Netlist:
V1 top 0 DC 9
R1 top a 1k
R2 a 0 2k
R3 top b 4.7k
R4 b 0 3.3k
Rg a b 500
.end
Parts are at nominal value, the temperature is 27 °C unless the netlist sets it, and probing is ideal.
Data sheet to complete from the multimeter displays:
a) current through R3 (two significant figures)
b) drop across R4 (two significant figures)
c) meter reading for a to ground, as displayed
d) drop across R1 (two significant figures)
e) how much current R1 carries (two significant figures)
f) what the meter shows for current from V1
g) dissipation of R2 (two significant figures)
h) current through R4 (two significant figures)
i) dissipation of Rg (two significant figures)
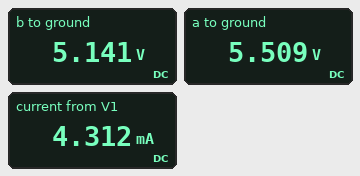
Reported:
820 µA
5.1 V
5.509 V
3.5 V
3.5 mA
4.312 mA
15 mW
1.6 mA
270 µW
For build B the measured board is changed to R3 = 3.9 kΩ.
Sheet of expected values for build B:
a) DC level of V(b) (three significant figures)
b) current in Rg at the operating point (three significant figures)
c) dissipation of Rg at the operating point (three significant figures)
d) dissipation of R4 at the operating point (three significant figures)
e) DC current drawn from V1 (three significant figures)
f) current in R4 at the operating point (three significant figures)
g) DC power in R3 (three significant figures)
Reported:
5.26 V
635 µA
201 µW
8.38 mW
4.38 mA
1.59 mA
3.59 mW
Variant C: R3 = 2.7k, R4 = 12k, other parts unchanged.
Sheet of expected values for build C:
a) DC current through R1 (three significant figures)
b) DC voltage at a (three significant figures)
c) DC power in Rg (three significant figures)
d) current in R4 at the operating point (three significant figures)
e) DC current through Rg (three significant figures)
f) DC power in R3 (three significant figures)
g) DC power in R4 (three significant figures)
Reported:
2.73 mA
6.27 V
79.8 µW
539 µA
400 µA
2.38 mW
3.48 mW
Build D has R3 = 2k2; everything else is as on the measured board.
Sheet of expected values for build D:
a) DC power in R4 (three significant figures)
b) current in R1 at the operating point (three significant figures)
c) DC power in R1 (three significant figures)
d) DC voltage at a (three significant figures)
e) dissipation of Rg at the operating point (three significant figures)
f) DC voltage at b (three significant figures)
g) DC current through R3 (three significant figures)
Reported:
9.91 mW
3.16 mA
9.99 mW
5.84 V
29.1 µW
5.72 V
1.49 mA
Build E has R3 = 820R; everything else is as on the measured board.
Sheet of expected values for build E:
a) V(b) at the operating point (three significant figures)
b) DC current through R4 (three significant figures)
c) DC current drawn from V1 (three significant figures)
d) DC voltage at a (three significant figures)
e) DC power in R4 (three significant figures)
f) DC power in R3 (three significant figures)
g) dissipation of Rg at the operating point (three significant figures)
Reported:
6.77 V
2.05 mA
5.27 mA
6.44 V
13.9 mW
6.05 mW
220 µW
